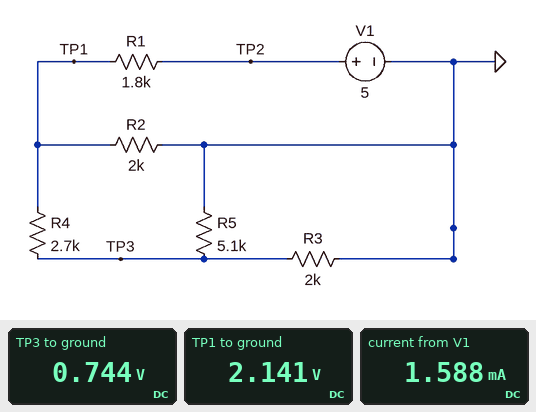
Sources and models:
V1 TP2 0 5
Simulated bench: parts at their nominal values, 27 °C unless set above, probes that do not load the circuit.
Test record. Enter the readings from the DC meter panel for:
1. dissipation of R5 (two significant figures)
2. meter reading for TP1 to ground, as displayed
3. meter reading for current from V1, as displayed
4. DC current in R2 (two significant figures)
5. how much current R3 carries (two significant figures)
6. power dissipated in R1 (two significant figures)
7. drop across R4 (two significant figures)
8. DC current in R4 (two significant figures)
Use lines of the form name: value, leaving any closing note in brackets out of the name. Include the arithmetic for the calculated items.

dissipation of R5: (744 mV)^2 / 5.1 kΩ = 110 µW
meter reading for TP1 to ground, as displayed: 2.141 V
meter reading for current from V1, as displayed: 1.588 mA
DC current in R2: (2.141 V) / 2 kΩ = 1.1 mA
how much current R3 carries: (744 mV) / 2 kΩ = 370 µA
power dissipated in R1: (5 V - 2.141 V)^2 / 1.8 kΩ = 4.5 mW
drop across R4: 2.141 V - 744 mV = 1.4 V
DC current in R4: (2.141 V - 744 mV) / 2.7 kΩ = 520 µA
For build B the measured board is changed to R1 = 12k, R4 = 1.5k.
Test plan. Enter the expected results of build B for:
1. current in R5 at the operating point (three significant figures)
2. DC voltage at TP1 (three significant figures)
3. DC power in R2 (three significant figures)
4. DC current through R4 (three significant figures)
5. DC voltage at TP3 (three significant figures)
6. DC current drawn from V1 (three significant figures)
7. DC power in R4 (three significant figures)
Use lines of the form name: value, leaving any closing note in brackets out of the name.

current in R5 at the operating point: 43.3 µA
DC voltage at TP1: 451 mV
DC power in R2: 102 µW
DC current through R4: 154 µA
DC voltage at TP3: 221 mV
DC current drawn from V1: 379 µA
DC power in R4: 35.4 µW
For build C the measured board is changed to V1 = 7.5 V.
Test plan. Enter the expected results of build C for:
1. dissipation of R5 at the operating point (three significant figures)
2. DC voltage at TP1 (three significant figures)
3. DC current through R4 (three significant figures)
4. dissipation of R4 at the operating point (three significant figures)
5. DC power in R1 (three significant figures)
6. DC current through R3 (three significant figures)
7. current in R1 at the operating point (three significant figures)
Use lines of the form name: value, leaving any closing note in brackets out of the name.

dissipation of R5 at the operating point: 244 µW
DC voltage at TP1: 3.21 V
DC current through R4: 776 µA
dissipation of R4 at the operating point: 1.63 mW
DC power in R1: 10.2 mW
DC current through R3: 558 µA
current in R1 at the operating point: 2.38 mA
